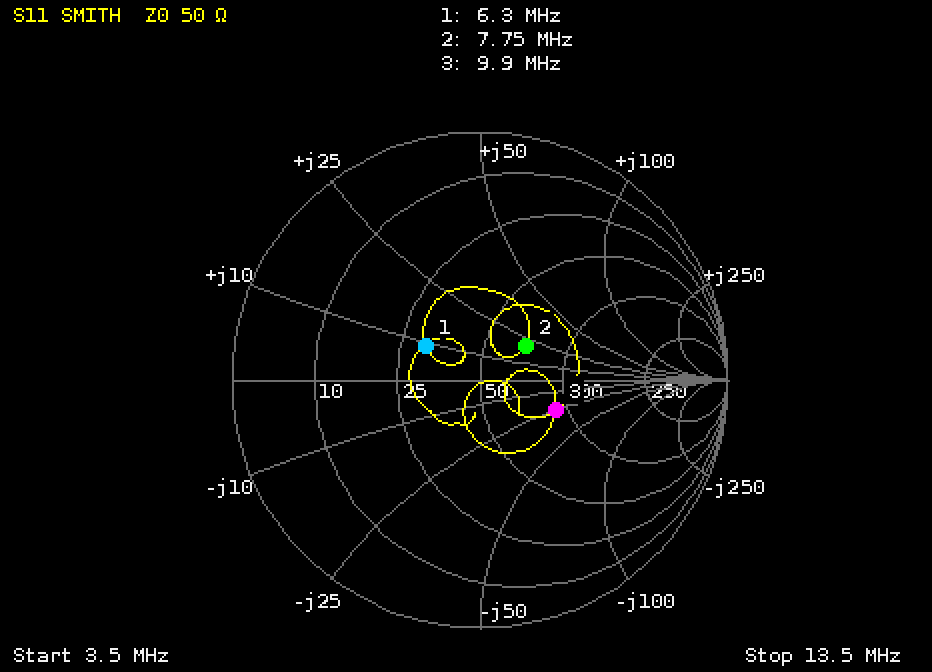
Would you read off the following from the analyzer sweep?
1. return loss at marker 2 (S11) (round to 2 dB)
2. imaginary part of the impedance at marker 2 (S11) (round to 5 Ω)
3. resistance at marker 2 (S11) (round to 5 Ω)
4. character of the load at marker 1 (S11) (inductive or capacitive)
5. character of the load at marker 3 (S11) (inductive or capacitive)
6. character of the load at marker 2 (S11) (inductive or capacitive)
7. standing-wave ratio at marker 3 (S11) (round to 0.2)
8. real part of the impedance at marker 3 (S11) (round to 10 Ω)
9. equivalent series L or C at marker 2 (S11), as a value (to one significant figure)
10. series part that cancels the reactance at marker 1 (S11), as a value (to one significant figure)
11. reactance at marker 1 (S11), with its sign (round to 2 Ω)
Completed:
12 dB
+20 Ω
70 Ω
inductive
capacitive
inductive
2.0
90 Ω
400 nH
3 nF
+10 Ω
